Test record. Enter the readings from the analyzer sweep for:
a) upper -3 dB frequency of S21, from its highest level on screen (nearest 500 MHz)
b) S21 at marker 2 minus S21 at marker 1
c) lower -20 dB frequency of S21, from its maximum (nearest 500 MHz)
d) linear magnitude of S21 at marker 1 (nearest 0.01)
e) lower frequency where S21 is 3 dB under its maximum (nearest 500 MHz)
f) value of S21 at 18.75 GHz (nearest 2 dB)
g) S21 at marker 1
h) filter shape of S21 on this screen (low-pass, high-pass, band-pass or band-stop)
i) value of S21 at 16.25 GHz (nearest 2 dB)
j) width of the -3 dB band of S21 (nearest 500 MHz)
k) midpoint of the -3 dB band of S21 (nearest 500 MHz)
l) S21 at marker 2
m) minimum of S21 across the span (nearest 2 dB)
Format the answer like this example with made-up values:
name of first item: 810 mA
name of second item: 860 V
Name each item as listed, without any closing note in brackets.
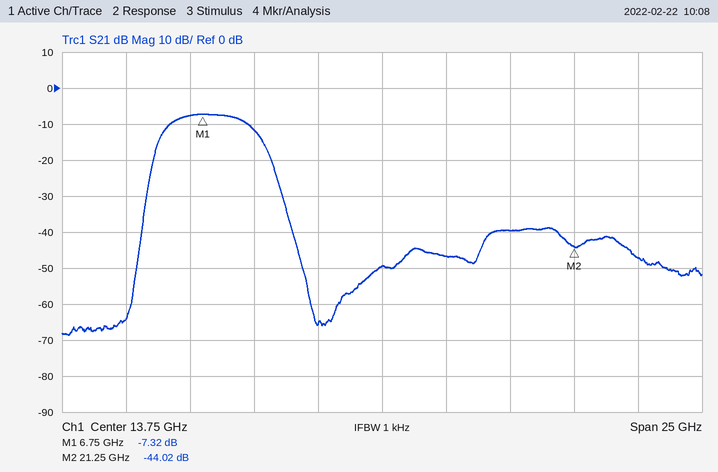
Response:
upper -3 dB frequency of S21, from its highest level on screen: 8.5 GHz
S21 at marker 2 minus S21 at marker 1: -36.70 dB
lower -20 dB frequency of S21, from its maximum: 4.5 GHz
linear magnitude of S21 at marker 1: 0.43
lower frequency where S21 is 3 dB under its maximum: 5.5 GHz
value of S21 at 18.75 GHz: -40 dB
S21 at marker 1: -7.32 dB
filter shape of S21 on this screen: band-pass
value of S21 at 16.25 GHz: -46 dB
width of the -3 dB band of S21: 3.0 GHz
midpoint of the -3 dB band of S21: 7.0 GHz
S21 at marker 2: -44.02 dB
minimum of S21 across the span: -68 dB
